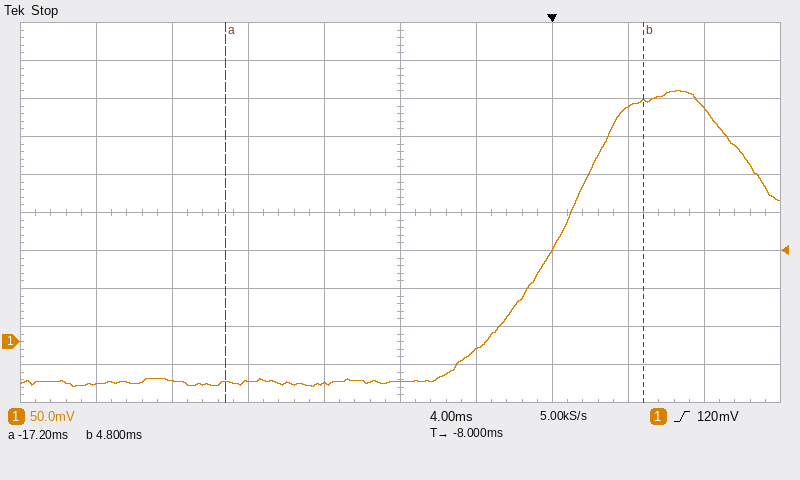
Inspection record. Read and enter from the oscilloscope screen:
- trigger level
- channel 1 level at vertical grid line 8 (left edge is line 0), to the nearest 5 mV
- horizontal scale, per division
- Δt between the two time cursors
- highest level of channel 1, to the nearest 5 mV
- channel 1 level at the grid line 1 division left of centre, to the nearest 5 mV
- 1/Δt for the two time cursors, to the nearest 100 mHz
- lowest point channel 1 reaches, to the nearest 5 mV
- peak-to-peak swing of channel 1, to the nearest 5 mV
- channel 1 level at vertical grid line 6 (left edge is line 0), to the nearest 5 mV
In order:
120 mV
310 mV
4 ms
22.0 ms
330 mV
-55 mV
45.5 Hz
-60 mV
390 mV
-10 mV
